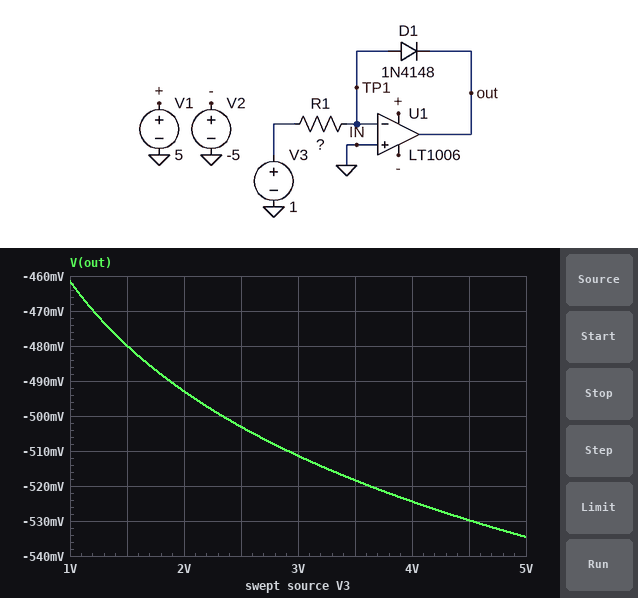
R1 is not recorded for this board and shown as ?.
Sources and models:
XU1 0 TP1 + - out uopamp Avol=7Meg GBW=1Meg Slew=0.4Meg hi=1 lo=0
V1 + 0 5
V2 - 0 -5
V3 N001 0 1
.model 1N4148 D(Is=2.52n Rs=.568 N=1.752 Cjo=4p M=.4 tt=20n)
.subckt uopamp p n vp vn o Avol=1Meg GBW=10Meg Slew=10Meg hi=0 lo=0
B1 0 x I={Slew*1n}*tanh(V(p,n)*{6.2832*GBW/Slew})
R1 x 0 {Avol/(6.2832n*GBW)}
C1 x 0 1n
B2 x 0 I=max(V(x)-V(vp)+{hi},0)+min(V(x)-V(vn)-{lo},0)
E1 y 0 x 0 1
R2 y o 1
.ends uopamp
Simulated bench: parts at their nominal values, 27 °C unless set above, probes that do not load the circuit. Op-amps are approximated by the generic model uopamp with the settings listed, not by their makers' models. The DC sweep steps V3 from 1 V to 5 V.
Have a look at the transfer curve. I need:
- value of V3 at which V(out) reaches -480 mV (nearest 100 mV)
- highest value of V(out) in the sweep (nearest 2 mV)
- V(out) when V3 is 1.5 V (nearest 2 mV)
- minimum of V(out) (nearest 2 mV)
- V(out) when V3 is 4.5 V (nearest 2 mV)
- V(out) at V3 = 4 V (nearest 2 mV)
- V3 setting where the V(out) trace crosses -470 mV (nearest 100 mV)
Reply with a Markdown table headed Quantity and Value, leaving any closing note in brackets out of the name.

| Quantity | Value |
|---|---|
| value of V3 at which V(out) reaches -480 mV | 1.5 V |
| highest value of V(out) in the sweep | -462 mV |
| V(out) when V3 is 1.5 V | -480 mV |
| minimum of V(out) | -534 mV |
| V(out) when V3 is 4.5 V | -530 mV |
| V(out) at V3 = 4 V | -524 mV |
| V3 setting where the V(out) trace crosses -470 mV | 1.2 V |
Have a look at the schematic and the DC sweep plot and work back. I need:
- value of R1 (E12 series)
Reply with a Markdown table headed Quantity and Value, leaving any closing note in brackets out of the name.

| Quantity | Value |
|---|---|
| value of R1 | 15 kΩ |
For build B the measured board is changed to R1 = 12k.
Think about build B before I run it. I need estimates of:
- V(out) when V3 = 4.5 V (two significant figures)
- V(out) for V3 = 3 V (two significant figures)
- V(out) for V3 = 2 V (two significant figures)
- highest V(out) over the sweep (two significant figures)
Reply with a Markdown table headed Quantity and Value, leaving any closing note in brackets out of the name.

| Quantity | Value |
|---|---|
| V(out) when V3 = 4.5 V | -540 mV |
| V(out) for V3 = 3 V | -520 mV |
| V(out) for V3 = 2 V | -500 mV |
| highest V(out) over the sweep | -470 mV |
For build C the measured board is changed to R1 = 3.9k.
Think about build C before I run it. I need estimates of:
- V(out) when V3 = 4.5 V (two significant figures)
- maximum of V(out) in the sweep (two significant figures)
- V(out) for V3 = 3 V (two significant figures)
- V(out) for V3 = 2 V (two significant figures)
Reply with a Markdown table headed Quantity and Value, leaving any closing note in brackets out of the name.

| Quantity | Value |
|---|---|
| V(out) when V3 = 4.5 V | -590 mV |
| maximum of V(out) in the sweep | -520 mV |
| V(out) for V3 = 3 V | -570 mV |
| V(out) for V3 = 2 V | -550 mV |
